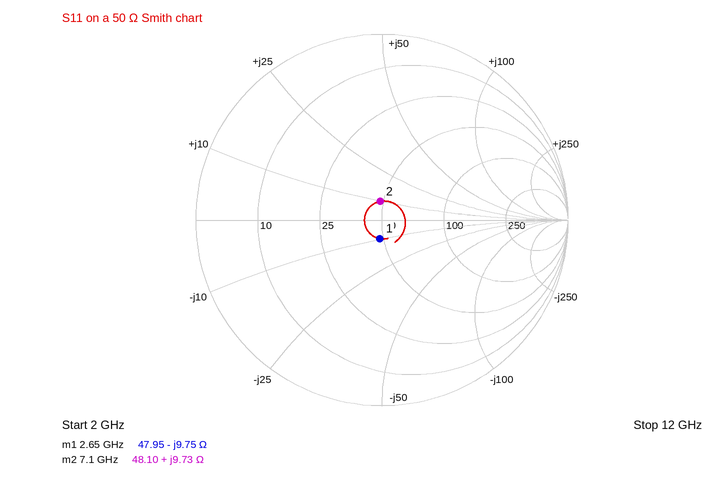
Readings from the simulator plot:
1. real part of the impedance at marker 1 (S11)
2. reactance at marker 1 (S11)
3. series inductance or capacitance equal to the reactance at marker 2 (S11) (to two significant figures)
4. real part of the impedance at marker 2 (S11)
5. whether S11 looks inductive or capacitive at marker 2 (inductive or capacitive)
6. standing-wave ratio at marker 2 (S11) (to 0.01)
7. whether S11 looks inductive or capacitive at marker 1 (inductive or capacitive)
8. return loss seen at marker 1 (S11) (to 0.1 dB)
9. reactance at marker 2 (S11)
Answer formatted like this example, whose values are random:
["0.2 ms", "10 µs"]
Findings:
["47.95 Ω", "-9.75 Ω", "220 pH", "48.10 Ω", "inductive", "1.22", "capacitive", "19.9 dB", "+9.73 Ω"]
